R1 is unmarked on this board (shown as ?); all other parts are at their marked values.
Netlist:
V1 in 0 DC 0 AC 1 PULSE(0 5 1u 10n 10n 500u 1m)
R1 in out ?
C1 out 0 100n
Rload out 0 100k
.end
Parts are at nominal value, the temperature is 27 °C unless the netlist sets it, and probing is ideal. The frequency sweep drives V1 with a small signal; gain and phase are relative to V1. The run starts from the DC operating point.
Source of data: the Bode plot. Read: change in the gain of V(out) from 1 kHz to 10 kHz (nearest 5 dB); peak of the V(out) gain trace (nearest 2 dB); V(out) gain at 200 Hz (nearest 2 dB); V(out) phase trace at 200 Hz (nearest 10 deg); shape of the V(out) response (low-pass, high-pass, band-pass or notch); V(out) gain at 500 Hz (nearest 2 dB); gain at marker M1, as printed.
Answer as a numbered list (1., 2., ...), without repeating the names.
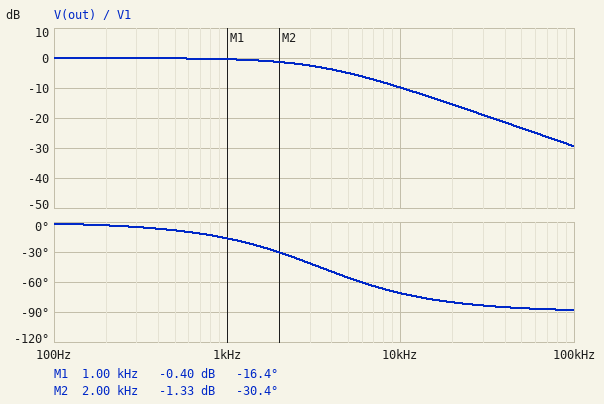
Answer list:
1. -10 dB
2. 0 dB
3. 0 dB
4. 0 deg
5. low-pass
6. 0 dB
7. -0.40 dB
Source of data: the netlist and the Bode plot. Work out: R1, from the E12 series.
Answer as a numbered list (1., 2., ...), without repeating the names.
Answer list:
1. 470 Ω
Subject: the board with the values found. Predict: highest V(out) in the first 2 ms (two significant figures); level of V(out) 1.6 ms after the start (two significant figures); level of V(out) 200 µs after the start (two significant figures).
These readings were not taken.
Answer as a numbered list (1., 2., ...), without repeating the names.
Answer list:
1. 5.0 V
2. 600 mV
3. 4.9 V
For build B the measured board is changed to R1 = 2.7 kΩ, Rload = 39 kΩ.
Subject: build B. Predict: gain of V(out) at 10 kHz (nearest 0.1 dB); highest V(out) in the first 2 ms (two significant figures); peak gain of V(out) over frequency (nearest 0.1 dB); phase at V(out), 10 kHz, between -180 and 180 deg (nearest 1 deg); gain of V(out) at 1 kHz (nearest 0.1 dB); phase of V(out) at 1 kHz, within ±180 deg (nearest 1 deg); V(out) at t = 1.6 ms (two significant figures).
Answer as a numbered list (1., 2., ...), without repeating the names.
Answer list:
1. -24.6 dB
2. 4.1 V
3. -0.6 dB
4. -86 deg
5. -6.0 dB
6. -58 deg
7. 2.8 V
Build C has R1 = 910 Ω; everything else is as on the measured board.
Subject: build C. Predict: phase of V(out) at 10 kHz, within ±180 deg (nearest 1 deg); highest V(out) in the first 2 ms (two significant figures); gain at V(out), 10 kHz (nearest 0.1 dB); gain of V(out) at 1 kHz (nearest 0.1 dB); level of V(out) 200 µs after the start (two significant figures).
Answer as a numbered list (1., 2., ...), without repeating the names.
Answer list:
1. -80 deg
2. 4.9 V
3. -15.3 dB
4. -1.3 dB
5. 4.4 V
